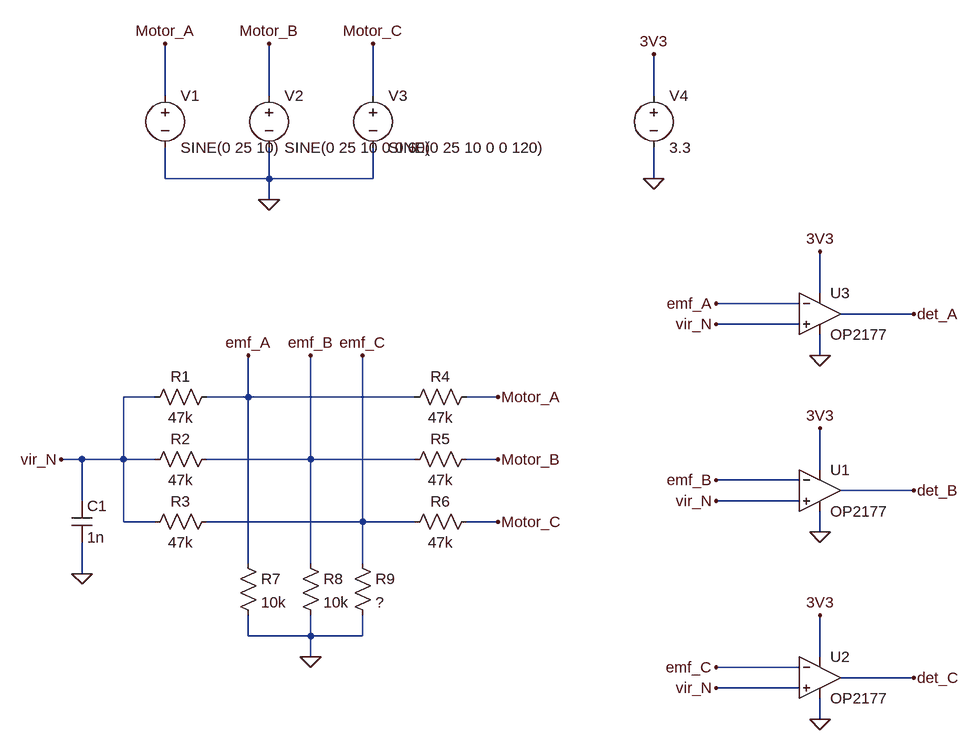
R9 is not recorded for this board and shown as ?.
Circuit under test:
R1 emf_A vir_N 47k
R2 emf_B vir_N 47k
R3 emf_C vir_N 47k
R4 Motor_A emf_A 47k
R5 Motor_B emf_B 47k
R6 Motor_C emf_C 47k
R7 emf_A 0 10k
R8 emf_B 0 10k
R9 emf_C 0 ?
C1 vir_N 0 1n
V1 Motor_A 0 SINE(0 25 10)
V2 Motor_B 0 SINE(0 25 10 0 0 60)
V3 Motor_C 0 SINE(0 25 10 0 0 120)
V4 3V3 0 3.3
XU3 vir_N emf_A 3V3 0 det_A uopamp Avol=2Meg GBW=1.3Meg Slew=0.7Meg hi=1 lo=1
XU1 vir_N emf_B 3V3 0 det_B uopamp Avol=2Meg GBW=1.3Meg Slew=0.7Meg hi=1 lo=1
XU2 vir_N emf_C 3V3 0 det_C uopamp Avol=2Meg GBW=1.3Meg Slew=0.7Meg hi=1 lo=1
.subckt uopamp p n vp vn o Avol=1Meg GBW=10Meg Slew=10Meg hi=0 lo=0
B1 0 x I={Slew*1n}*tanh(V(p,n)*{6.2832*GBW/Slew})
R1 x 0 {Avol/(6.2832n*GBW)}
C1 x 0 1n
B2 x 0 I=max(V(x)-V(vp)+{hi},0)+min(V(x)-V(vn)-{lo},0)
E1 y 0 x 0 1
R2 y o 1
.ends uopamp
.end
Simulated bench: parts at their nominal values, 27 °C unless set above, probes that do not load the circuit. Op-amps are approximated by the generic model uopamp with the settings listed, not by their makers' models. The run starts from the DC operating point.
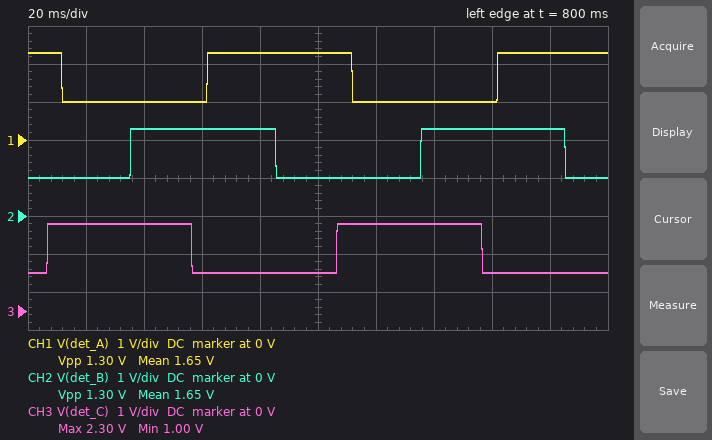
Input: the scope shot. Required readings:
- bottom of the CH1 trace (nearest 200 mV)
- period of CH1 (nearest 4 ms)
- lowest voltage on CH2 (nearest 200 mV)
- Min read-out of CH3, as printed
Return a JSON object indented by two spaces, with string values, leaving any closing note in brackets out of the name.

{
  "bottom of the CH1 trace": "1.0 V",
  "period of CH1": "100 ms",
  "lowest voltage on CH2": "1.0 V",
  "Min read-out of CH3, as printed": "1.00 V"
}
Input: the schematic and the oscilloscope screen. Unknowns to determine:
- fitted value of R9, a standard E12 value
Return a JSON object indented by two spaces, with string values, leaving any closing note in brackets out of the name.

{
  "fitted value of R9, a standard E12 value": "12 kΩ"
}
